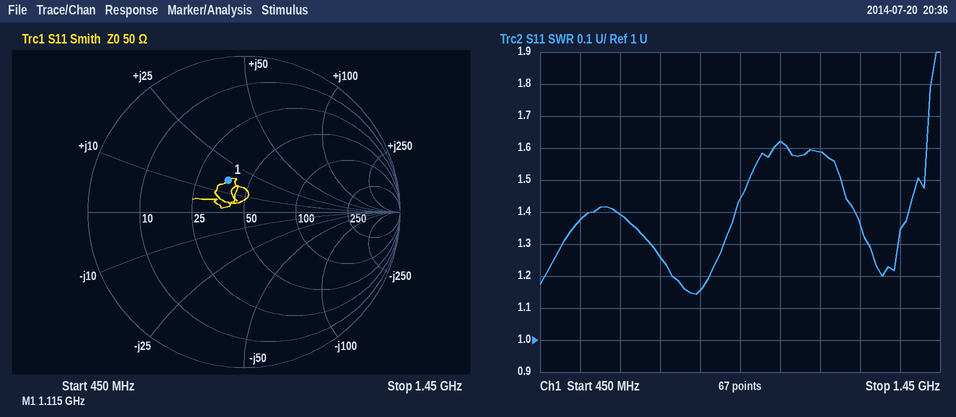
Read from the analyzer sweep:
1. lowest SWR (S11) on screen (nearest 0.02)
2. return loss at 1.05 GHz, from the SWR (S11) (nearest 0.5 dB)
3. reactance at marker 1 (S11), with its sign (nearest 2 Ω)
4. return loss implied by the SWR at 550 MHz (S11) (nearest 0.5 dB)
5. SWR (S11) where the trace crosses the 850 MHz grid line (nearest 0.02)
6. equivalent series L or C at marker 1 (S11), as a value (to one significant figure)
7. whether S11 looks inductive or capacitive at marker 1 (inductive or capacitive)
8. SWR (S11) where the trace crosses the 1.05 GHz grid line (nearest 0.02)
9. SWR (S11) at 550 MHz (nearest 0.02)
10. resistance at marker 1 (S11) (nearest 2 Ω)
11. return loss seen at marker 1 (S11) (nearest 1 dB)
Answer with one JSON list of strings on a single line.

["1.14", "12.5 dB", "+16 Ω", "16.0 dB", "1.16", "2 nH", "inductive", "1.62", "1.38", "38 Ω", "13 dB"]
